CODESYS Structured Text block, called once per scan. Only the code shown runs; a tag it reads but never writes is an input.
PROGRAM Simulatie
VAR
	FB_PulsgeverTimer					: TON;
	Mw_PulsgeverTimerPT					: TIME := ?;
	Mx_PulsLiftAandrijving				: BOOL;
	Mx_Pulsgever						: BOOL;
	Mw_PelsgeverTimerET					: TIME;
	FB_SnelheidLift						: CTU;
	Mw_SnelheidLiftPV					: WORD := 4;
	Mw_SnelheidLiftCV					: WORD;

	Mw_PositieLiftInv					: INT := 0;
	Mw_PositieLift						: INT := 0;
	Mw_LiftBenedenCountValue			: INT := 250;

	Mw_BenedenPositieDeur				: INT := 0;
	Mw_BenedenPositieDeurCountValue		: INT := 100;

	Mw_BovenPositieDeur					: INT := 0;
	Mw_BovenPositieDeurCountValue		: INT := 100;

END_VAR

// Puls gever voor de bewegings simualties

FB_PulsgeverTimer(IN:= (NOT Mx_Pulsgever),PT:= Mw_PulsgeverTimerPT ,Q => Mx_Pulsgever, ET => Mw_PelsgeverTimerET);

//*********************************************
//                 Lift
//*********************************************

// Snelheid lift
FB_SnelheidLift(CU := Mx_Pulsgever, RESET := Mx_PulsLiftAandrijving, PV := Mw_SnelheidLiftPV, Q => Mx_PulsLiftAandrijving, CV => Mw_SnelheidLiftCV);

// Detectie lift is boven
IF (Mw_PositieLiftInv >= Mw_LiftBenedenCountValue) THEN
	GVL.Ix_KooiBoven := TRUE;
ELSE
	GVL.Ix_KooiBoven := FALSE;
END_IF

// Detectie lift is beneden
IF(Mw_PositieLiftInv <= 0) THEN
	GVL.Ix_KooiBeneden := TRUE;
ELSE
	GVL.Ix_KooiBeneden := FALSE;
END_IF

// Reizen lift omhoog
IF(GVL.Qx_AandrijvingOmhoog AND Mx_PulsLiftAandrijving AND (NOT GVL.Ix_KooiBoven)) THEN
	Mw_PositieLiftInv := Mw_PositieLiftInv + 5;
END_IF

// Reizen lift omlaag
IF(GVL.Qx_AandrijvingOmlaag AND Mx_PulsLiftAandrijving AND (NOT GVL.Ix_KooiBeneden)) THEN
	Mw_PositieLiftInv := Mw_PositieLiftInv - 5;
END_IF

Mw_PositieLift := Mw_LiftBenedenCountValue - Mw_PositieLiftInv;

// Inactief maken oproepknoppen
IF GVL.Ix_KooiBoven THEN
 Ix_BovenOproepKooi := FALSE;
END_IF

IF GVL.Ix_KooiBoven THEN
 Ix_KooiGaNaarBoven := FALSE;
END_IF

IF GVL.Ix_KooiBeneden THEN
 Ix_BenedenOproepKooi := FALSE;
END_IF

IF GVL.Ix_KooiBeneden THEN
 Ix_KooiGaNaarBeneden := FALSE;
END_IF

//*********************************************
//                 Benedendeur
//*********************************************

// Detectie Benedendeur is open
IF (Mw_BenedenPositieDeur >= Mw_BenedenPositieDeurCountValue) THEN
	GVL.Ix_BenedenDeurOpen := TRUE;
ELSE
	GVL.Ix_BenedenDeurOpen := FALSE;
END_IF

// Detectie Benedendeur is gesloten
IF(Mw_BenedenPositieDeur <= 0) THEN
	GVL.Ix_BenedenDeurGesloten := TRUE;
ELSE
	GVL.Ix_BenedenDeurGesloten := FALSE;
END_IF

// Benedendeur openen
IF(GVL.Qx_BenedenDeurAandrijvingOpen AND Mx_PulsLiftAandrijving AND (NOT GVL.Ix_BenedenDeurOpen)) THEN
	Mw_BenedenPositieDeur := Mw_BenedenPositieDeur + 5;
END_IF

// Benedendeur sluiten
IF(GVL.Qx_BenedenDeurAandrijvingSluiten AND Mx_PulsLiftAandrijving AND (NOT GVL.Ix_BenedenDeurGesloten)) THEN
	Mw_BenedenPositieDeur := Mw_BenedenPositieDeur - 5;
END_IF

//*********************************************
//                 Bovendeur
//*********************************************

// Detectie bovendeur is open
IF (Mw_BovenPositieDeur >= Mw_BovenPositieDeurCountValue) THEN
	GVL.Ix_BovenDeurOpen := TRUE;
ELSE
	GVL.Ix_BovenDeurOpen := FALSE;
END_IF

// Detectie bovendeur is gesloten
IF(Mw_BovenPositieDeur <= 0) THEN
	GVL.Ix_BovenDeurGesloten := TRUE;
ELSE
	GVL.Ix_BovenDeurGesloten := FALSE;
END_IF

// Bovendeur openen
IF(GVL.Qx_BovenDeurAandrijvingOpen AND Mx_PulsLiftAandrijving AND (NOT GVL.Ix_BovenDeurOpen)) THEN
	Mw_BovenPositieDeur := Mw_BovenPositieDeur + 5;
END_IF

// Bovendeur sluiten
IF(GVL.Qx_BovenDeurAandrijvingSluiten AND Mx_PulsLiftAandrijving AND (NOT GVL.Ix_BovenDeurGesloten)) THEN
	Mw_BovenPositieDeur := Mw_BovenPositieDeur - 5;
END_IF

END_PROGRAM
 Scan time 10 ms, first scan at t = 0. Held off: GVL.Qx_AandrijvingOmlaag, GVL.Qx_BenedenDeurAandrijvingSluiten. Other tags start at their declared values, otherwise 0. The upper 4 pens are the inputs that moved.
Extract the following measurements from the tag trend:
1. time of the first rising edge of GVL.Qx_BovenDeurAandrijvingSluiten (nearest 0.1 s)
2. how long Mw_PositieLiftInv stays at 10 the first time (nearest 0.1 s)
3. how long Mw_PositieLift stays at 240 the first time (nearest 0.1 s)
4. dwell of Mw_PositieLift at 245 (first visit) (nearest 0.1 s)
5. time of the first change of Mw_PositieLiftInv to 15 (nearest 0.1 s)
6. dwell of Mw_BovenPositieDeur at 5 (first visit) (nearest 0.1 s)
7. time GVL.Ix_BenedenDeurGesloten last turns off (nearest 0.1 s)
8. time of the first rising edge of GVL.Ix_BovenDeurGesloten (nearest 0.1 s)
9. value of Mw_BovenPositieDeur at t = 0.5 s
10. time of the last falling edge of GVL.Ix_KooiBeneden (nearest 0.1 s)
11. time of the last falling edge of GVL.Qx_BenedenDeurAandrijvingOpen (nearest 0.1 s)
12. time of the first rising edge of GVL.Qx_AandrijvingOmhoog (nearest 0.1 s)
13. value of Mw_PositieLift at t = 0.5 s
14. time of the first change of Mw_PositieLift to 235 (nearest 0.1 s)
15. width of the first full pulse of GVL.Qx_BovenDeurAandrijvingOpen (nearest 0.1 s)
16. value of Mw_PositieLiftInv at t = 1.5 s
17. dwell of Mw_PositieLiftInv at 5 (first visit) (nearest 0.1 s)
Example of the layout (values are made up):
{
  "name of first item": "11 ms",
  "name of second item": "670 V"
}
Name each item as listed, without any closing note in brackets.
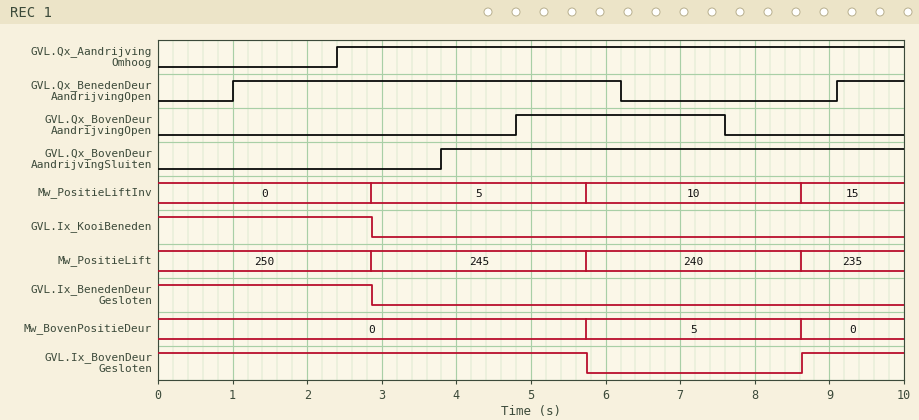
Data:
{
  "time of the first rising edge of GVL.Qx_BovenDeurAandrijvingSluiten": "3.8 s",
  "how long Mw_PositieLiftInv stays at 10 the first time": "2.9 s",
  "how long Mw_PositieLift stays at 240 the first time": "2.9 s",
  "dwell of Mw_PositieLift at 245 (first visit)": "2.9 s",
  "time of the first change of Mw_PositieLiftInv to 15": "8.6 s",
  "dwell of Mw_BovenPositieDeur at 5 (first visit)": "2.9 s",
  "time GVL.Ix_BenedenDeurGesloten last turns off": "2.9 s",
  "time of the first rising edge of GVL.Ix_BovenDeurGesloten": "8.6 s",
  "value of Mw_BovenPositieDeur at t = 0.5 s": "0",
  "time of the last falling edge of GVL.Ix_KooiBeneden": "2.9 s",
  "time of the last falling edge of GVL.Qx_BenedenDeurAandrijvingOpen": "6.2 s",
  "time of the first rising edge of GVL.Qx_AandrijvingOmhoog": "2.4 s",
  "value of Mw_PositieLift at t = 0.5 s": "250",
  "time of the first change of Mw_PositieLift to 235": "8.6 s",
  "width of the first full pulse of GVL.Qx_BovenDeurAandrijvingOpen": "2.8 s",
  "value of Mw_PositieLiftInv at t = 1.5 s": "0",
  "dwell of Mw_PositieLiftInv at 5 (first visit)": "2.9 s"
}
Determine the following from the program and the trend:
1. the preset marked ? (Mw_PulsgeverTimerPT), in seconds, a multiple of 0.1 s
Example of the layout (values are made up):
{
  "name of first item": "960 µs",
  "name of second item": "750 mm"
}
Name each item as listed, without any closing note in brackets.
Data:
{
  "the preset marked ? (Mw_PulsgeverTimerPT), in seconds, a multiple of 0.1 s": "0.7 s"
}
